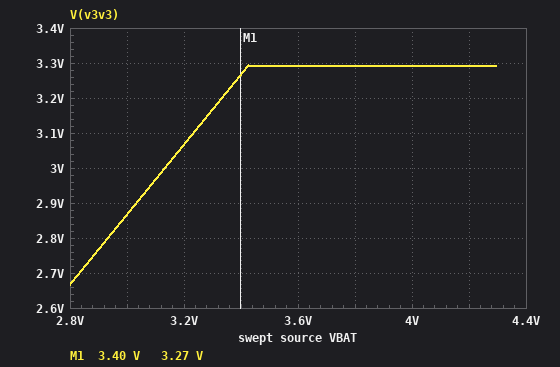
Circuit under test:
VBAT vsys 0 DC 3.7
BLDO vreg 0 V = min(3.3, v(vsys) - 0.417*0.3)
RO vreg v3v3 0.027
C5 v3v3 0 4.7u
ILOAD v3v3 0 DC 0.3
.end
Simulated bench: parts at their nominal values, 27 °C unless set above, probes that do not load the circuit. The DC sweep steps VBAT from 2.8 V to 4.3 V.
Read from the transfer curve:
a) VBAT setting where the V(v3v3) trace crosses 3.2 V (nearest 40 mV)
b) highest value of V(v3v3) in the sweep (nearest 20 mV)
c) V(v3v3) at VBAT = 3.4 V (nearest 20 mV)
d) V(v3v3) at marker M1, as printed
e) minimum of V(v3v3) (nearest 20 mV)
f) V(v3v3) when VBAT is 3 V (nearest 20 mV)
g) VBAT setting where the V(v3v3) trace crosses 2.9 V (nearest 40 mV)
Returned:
3.32 V
3.30 V
3.26 V
3.27 V
2.66 V
2.86 V
3.04 V
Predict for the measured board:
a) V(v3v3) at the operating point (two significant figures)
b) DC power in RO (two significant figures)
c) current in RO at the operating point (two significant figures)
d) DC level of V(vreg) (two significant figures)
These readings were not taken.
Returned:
3.3 V
2.4 mW
300 mA
3.3 V
